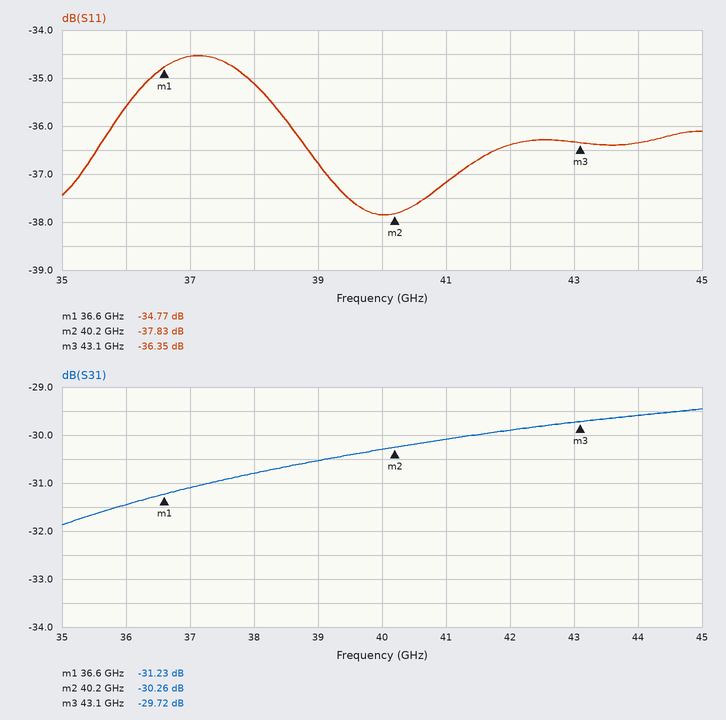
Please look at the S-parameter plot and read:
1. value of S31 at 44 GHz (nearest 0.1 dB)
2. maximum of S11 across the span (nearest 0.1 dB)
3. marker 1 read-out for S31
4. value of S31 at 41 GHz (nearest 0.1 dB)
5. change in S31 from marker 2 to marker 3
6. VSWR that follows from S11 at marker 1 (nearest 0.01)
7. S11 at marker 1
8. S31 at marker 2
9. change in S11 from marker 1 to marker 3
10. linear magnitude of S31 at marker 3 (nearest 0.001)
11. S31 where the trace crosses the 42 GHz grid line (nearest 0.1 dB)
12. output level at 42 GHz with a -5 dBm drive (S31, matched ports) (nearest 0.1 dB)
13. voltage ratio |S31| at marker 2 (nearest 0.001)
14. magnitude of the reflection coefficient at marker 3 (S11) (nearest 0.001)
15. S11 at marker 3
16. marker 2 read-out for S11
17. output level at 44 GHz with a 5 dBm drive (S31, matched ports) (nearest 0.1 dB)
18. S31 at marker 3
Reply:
-29.6 dB
-34.5 dB
-31.23 dB
-30.1 dB
0.54 dB
1.04
-34.77 dB
-30.26 dB
-1.58 dB
0.033
-29.9 dB
-34.9 dBm
0.031
0.015
-36.35 dB
-37.83 dB
-24.6 dBm
-29.72 dB
